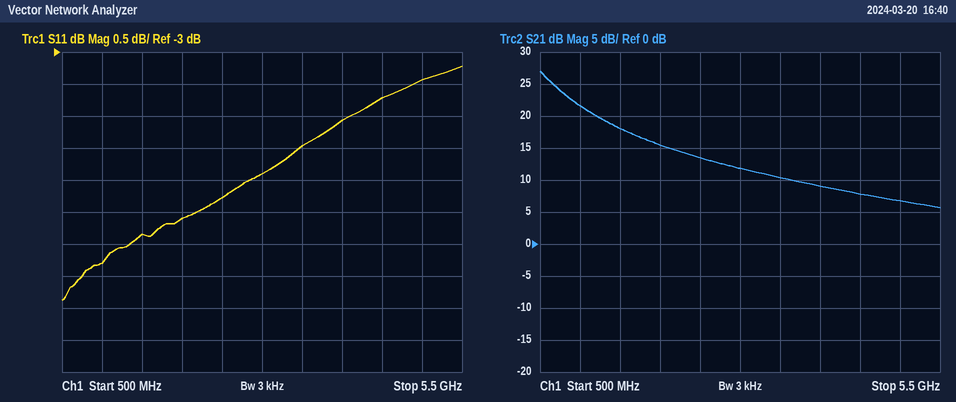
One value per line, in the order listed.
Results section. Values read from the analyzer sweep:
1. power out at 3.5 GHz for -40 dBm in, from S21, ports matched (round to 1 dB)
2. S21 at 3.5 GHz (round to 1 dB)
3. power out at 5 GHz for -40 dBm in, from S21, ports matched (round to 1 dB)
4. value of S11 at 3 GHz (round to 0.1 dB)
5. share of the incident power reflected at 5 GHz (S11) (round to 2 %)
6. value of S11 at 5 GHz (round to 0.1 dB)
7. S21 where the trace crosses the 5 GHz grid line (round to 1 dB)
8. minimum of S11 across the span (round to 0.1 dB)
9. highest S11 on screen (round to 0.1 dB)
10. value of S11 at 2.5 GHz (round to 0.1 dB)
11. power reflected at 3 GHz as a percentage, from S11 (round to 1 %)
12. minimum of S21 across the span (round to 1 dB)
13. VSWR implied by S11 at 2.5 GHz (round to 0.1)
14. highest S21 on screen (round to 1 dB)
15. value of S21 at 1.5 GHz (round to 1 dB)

-30 dBm
10 dB
-33 dBm
-4.9 dB
46 %
-3.4 dB
7 dB
-6.9 dB
-3.2 dB
-5.3 dB
32 %
6 dB
3.4
27 dB
18 dB
